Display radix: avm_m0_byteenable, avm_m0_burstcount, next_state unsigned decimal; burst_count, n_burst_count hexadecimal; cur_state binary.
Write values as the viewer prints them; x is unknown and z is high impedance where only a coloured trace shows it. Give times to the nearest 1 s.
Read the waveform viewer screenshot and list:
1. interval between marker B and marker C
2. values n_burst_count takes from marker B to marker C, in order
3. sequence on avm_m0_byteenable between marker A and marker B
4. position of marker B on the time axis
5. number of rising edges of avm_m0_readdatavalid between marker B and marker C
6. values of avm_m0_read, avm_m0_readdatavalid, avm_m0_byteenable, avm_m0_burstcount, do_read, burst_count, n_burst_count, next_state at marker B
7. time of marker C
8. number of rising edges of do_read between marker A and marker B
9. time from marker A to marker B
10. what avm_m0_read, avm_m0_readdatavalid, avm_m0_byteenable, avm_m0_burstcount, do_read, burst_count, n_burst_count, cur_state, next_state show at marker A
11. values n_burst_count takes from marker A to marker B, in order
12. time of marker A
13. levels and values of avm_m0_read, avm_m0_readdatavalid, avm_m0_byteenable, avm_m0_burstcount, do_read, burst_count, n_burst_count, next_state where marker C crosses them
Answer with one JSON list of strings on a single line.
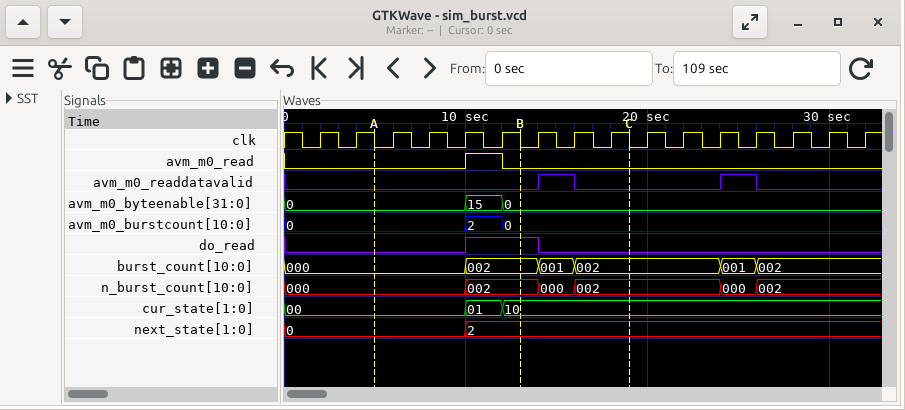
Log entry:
["6 s", "002, 000, 002", "0, 15, 0", "13 s", "1", "avm_m0_read=0, avm_m0_readdatavalid=0, avm_m0_byteenable=0, avm_m0_burstcount=0, do_read=1, burst_count=002, n_burst_count=002, next_state=2", "19 s", "1", "8 s", "avm_m0_read=0, avm_m0_readdatavalid=0, avm_m0_byteenable=0, avm_m0_burstcount=0, do_read=0, burst_count=000, n_burst_count=000, cur_state=00, next_state=0", "000, 002", "5 s", "avm_m0_read=0, avm_m0_readdatavalid=0, avm_m0_byteenable=0, avm_m0_burstcount=0, do_read=0, burst_count=002, n_burst_count=002, next_state=2"]
